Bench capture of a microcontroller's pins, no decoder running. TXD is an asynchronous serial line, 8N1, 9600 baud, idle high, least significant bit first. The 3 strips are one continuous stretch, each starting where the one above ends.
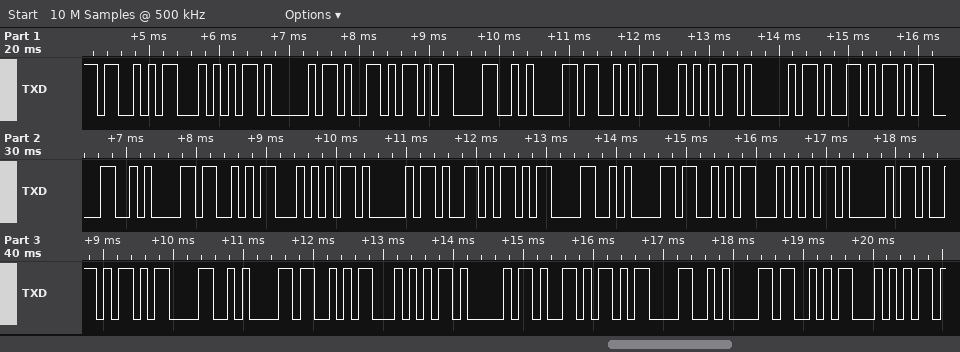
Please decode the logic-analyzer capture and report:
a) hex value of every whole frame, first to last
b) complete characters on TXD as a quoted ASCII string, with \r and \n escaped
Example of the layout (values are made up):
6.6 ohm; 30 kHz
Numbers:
53 54 41 59 0D 0A 53 54 41 59 0D 0A 53 54 41 59 0D 0A 53 54 41 59 0D 0A 53 54 41 59 0D 0A 53 54; "STAY\r\nSTAY\r\nSTAY\r\nSTAY\r\nSTAY\r\nST"
